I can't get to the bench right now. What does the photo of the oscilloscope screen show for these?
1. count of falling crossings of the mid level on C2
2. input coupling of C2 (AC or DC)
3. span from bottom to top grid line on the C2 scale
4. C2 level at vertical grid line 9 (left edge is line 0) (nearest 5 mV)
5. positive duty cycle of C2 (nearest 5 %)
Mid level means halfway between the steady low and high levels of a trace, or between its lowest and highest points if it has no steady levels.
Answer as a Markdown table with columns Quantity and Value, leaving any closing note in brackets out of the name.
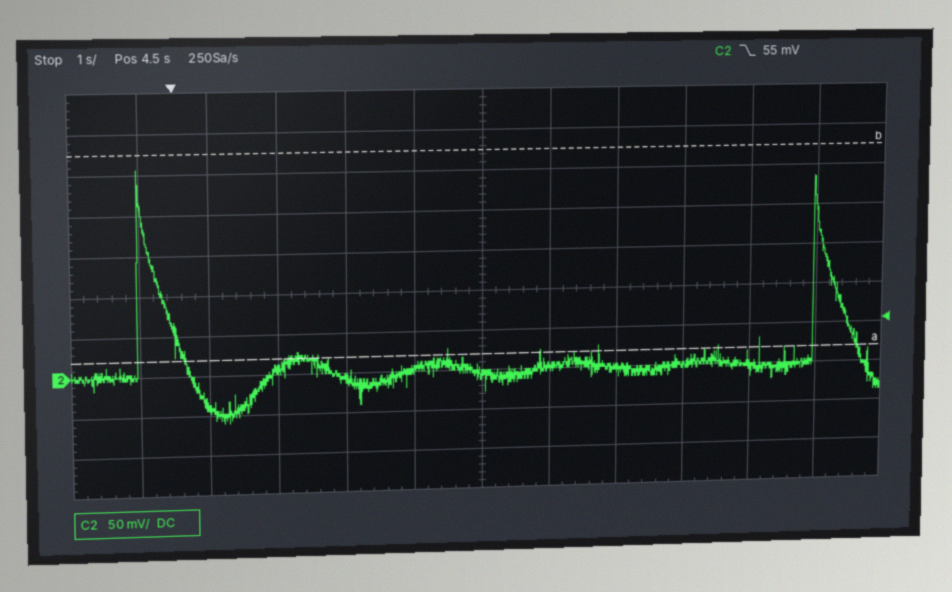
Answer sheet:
| Quantity | Value |
|---|---|
| count of falling crossings of the mid level on C2 | 2 |
| input coupling of C2 | DC |
| span from bottom to top grid line on the C2 scale | 500 mV |
| C2 level at vertical grid line 9 (left edge is line 0) | 0 mV |
| positive duty cycle of C2 | 5 % |
